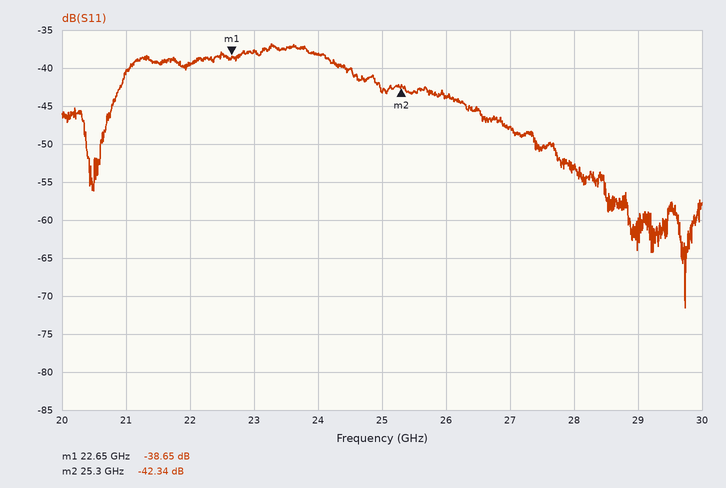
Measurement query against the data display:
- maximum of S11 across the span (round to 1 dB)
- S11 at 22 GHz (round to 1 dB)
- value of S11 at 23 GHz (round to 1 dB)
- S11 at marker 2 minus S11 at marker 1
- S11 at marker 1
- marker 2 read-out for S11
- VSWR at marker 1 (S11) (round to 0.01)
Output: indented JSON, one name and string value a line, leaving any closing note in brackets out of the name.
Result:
{
  "maximum of S11 across the span": "-37 dB",
  "S11 at 22 GHz": "-39 dB",
  "value of S11 at 23 GHz": "-38 dB",
  "S11 at marker 2 minus S11 at marker 1": "-3.69 dB",
  "S11 at marker 1": "-38.65 dB",
  "marker 2 read-out for S11": "-42.34 dB",
  "VSWR at marker 1 (S11)": "1.02"
}
